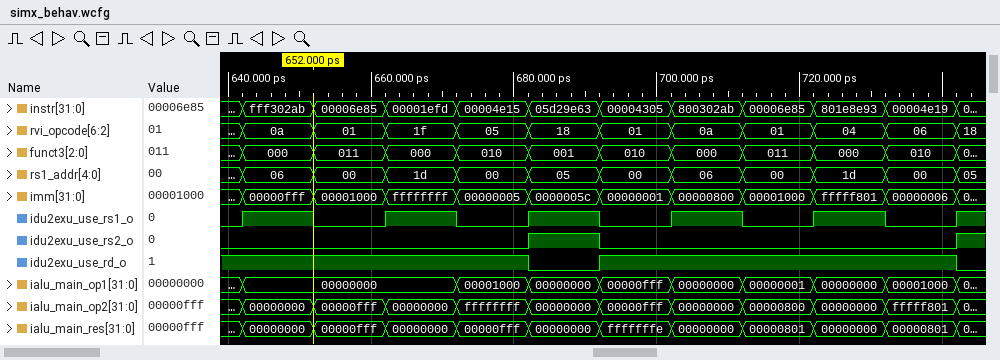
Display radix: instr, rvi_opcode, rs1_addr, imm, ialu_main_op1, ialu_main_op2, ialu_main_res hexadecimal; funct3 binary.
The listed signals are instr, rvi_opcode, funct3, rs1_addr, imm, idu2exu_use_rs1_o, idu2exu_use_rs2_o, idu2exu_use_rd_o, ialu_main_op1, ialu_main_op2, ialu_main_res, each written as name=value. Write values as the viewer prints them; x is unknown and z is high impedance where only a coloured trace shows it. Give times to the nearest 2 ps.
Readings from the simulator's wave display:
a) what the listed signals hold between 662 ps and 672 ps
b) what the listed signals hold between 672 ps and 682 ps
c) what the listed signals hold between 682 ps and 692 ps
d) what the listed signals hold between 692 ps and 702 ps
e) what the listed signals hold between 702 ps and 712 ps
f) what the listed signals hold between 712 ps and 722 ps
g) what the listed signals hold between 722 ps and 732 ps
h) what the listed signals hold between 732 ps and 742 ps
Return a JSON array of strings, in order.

["instr=00001efd, rvi_opcode=1f, funct3=000, rs1_addr=1d, imm=ffffffff, idu2exu_use_rs1_o=1, idu2exu_use_rs2_o=0, idu2exu_use_rd_o=1, ialu_main_op1=00000000, ialu_main_op2=00000000, ialu_main_res=00000000", "instr=00004e15, rvi_opcode=05, funct3=010, rs1_addr=00, imm=00000005, idu2exu_use_rs1_o=0, idu2exu_use_rs2_o=0, idu2exu_use_rd_o=1, ialu_main_op1=00001000, ialu_main_op2=ffffffff, ialu_main_res=00000fff", "instr=05d29e63, rvi_opcode=18, funct3=001, rs1_addr=05, imm=0000005c, idu2exu_use_rs1_o=1, idu2exu_use_rs2_o=1, idu2exu_use_rd_o=0, ialu_main_op1=00000000, ialu_main_op2=00000000, ialu_main_res=00000000", "instr=00004305, rvi_opcode=01, funct3=010, rs1_addr=00, imm=00000001, idu2exu_use_rs1_o=0, idu2exu_use_rs2_o=0, idu2exu_use_rd_o=1, ialu_main_op1=00000fff, ialu_main_op2=00000fff, ialu_main_res=fffffffe", "instr=800302ab, rvi_opcode=0a, funct3=000, rs1_addr=06, imm=00000800, idu2exu_use_rs1_o=1, idu2exu_use_rs2_o=0, idu2exu_use_rd_o=1, ialu_main_op1=00000000, ialu_main_op2=00000000, ialu_main_res=00000000", "instr=00006e85, rvi_opcode=01, funct3=011, rs1_addr=00, imm=00001000, idu2exu_use_rs1_o=0, idu2exu_use_rs2_o=0, idu2exu_use_rd_o=1, ialu_main_op1=00000001, ialu_main_op2=00000800, ialu_main_res=00000801", "instr=801e8e93, rvi_opcode=04, funct3=000, rs1_addr=1d, imm=fffff801, idu2exu_use_rs1_o=1, idu2exu_use_rs2_o=0, idu2exu_use_rd_o=1, ialu_main_op1=00000000, ialu_main_op2=00000000, ialu_main_res=00000000", "instr=00004e19, rvi_opcode=06, funct3=010, rs1_addr=00, imm=00000006, idu2exu_use_rs1_o=0, idu2exu_use_rs2_o=0, idu2exu_use_rd_o=1, ialu_main_op1=00001000, ialu_main_op2=fffff801, ialu_main_res=00000801"]
